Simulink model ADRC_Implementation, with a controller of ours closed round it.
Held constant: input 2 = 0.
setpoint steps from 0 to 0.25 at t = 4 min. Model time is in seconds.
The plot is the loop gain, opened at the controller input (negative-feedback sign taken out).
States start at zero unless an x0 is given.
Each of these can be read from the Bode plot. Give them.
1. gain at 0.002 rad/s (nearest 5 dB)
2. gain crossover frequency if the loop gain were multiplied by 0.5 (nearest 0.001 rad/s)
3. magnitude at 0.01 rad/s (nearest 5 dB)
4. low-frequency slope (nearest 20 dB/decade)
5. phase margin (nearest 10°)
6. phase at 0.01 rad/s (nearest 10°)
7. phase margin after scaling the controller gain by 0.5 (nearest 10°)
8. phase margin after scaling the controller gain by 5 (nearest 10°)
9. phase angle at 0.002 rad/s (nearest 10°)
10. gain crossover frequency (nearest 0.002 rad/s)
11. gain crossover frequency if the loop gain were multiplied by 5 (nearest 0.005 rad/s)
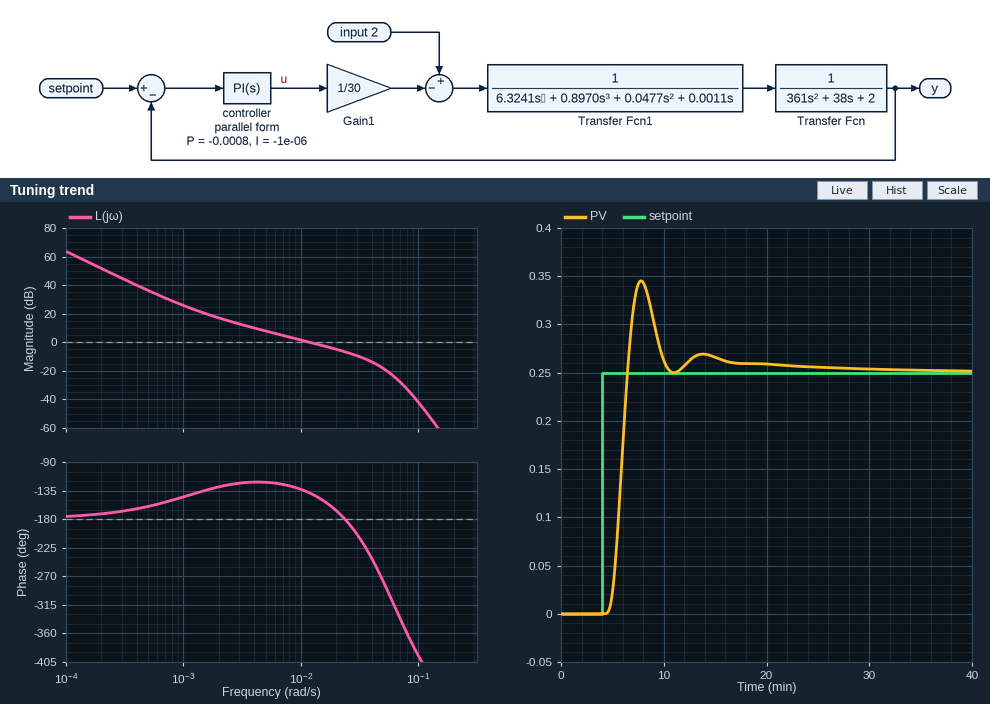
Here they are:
15 dB
0.006 rad/s
0 dB
-40 dB/decade
40°
-130°
60°
-60°
-130°
0.012 rad/s
0.040 rad/s
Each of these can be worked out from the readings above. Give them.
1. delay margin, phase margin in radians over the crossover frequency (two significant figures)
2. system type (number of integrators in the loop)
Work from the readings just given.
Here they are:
58 s
2
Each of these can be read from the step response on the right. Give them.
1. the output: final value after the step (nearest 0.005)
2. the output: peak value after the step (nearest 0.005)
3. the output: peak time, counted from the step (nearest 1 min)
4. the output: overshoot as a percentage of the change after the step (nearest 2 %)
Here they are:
0.250
0.345
4 min
38 %
